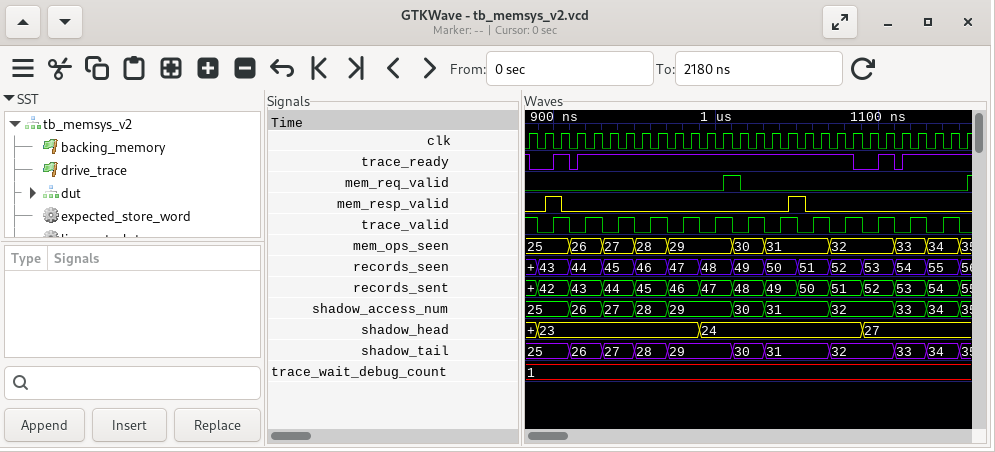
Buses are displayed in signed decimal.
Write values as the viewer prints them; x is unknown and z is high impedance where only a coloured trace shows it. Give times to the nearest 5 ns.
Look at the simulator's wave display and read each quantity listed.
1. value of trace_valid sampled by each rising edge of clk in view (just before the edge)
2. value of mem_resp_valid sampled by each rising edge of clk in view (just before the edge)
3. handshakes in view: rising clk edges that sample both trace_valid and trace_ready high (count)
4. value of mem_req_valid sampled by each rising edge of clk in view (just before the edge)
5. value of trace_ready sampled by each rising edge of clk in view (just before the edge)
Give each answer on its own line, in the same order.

1 0 1 0 1 0 1 0 1 0 1 0 1 0 1 0 1 0 1 0 1 0 1 0 1 0 1 0
0 0 1 0 0 0 0 0 0 0 0 0 0 0 0 0 0 1 0 0 0 0 0 0 0 0 0 0
14
0 0 0 0 0 0 0 0 0 0 0 0 0 1 0 0 0 0 0 0 0 0 0 0 0 0 0 0
1 0 1 0 1 1 1 1 1 1 1 1 1 1 1 1 1 1 1 1 1 0 1 0 1 1 1 1
